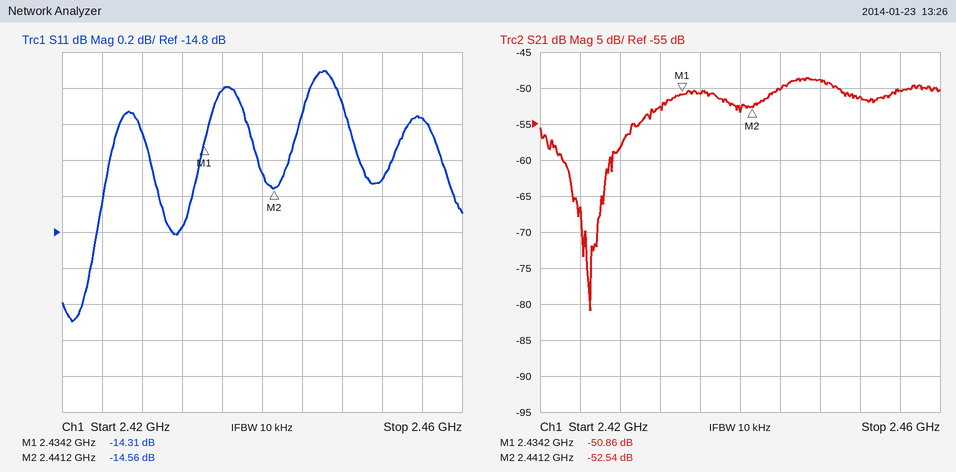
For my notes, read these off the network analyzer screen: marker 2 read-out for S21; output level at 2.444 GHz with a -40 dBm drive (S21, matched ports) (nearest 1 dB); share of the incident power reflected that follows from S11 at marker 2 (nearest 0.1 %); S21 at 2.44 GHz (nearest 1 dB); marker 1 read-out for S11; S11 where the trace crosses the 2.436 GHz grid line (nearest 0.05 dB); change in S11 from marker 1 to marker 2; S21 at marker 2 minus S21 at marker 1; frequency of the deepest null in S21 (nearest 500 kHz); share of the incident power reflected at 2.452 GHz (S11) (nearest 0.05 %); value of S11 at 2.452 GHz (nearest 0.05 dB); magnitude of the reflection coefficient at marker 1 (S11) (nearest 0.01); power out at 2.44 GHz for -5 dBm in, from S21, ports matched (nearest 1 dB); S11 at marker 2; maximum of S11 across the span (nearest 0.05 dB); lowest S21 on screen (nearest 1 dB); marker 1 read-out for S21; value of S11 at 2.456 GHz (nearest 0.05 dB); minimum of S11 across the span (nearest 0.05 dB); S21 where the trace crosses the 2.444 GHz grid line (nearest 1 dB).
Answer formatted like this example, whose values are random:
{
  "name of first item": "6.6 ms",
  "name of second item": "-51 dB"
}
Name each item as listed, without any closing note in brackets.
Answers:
{
  "marker 2 read-out for S21": "-52.54 dB",
  "output level at 2.444 GHz with a -40 dBm drive (S21, matched ports)": "-90 dBm",
  "share of the incident power reflected that follows from S11 at marker 2": "3.5 %",
  "S21 at 2.44 GHz": "-53 dB",
  "marker 1 read-out for S11": "-14.31 dB",
  "S11 where the trace crosses the 2.436 GHz grid line": "-14.00 dB",
  "change in S11 from marker 1 to marker 2": "-0.25 dB",
  "S21 at marker 2 minus S21 at marker 1": "-1.68 dB",
  "frequency of the deepest null in S21": "2.4250 GHz",
  "share of the incident power reflected at 2.452 GHz (S11)": "3.55 %",
  "value of S11 at 2.452 GHz": "-14.50 dB",
  "magnitude of the reflection coefficient at marker 1 (S11)": "0.19",
  "power out at 2.44 GHz for -5 dBm in, from S21, ports matched": "-58 dBm",
  "S11 at marker 2": "-14.56 dB",
  "maximum of S11 across the span": "-13.90 dB",
  "lowest S21 on screen": "-81 dB",
  "marker 1 read-out for S21": "-50.86 dB",
  "value of S11 at 2.456 GHz": "-14.15 dB",
  "minimum of S11 across the span": "-15.30 dB",
  "S21 where the trace crosses the 2.444 GHz grid line": "-50 dB"
}
